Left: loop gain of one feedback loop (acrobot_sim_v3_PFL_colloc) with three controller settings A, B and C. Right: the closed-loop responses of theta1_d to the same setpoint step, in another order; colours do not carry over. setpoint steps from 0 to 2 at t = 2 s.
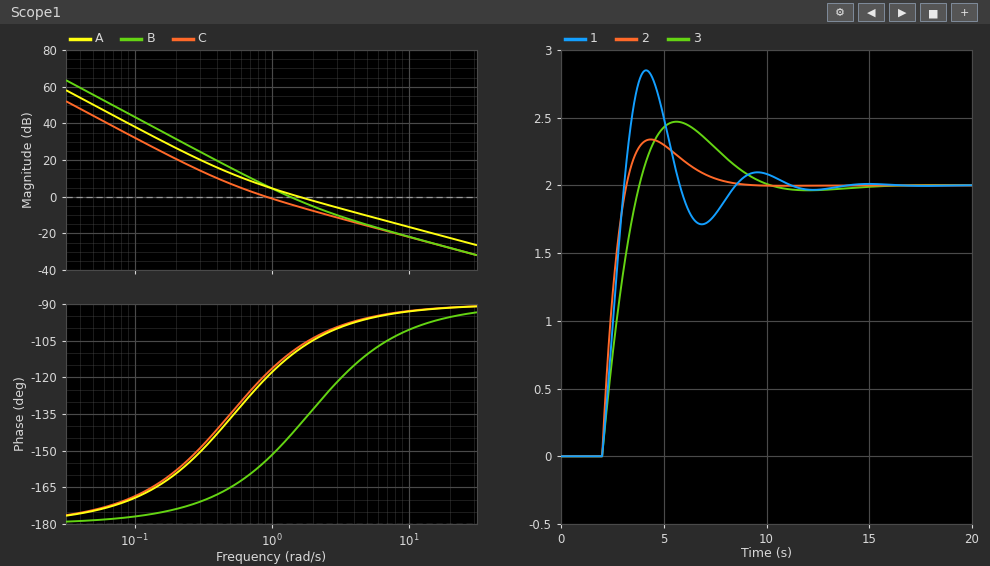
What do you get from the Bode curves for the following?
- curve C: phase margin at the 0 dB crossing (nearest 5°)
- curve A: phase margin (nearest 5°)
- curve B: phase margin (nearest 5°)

60°
70°
35°
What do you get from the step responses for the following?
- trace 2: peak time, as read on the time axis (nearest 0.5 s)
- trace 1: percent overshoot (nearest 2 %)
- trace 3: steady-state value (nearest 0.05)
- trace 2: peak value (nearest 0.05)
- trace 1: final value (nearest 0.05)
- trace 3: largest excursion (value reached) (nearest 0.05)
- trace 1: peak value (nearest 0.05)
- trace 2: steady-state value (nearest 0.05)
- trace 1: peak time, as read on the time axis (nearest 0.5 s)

4.5 s
42 %
2.00
2.35
2.00
2.45
2.85
2.00
4.0 s
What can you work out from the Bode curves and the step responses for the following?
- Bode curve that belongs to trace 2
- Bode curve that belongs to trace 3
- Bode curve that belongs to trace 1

A
C
B
